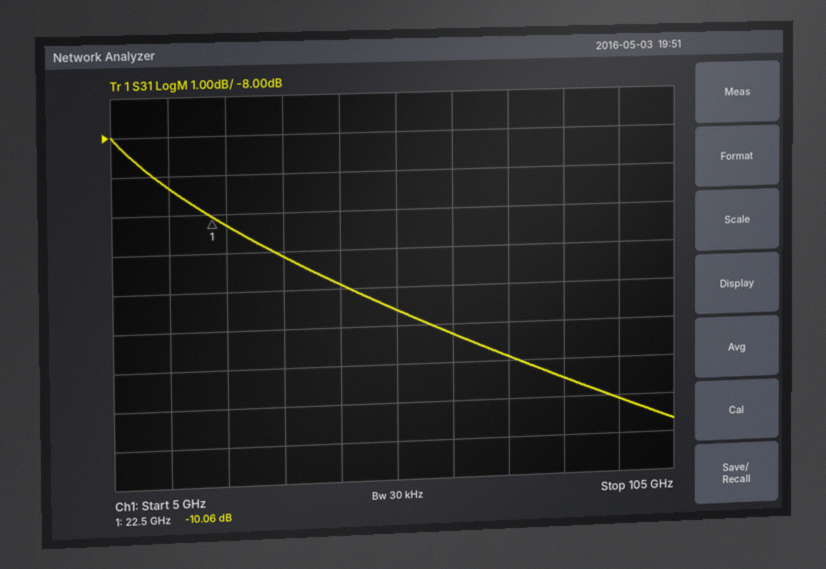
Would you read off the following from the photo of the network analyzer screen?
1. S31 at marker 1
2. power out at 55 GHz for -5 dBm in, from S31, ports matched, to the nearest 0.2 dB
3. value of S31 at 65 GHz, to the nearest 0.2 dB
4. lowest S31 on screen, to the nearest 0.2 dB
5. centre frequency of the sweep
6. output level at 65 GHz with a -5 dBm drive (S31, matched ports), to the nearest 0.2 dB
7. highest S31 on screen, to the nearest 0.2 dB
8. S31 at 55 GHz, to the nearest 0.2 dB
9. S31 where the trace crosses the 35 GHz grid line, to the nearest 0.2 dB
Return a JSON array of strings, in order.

["-10.06 dB", "-17.6 dBm", "-13.2 dB", "-15.6 dB", "55 GHz", "-18.2 dBm", "-8.0 dB", "-12.6 dB", "-11.2 dB"]
